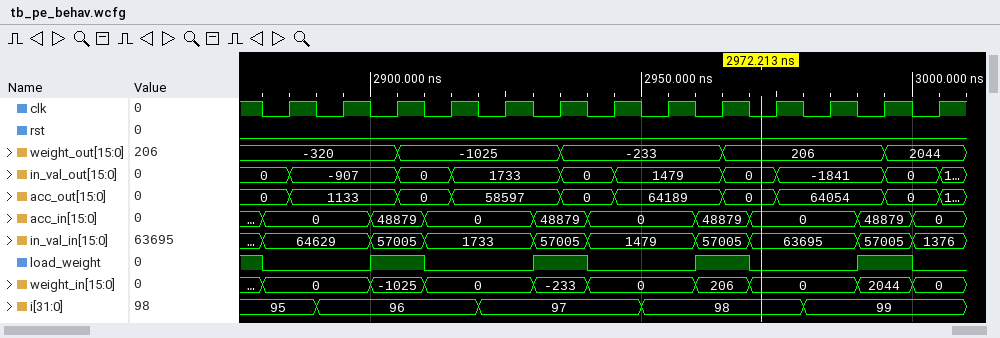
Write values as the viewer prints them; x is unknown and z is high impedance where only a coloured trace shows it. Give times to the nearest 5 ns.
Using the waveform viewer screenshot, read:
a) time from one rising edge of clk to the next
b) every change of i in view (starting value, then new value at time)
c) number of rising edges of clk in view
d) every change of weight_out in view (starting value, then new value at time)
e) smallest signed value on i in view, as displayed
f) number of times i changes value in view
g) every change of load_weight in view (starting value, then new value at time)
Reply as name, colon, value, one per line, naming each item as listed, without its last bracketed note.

time from one rising edge of clk to the next: 10 ns
every change of i in view: 95, 96 at 2890 ns, 97 at 2920 ns, 98 at 2950 ns, 99 at 2980 ns
number of rising edges of clk in view: 13
every change of weight_out in view: -320, -1025 at 2905 ns, -233 at 2935 ns, 206 at 2965 ns, 2044 at 2995 ns
smallest signed value on i in view, as displayed: 95
number of times i changes value in view: 4
every change of load_weight in view: 1, 0 at 2880 ns, 1 at 2900 ns, 0 at 2910 ns, 1 at 2930 ns, 0 at 2940 ns, 1 at 2960 ns, 0 at 2970 ns, 1 at 2990 ns, 0 at 3000 ns
